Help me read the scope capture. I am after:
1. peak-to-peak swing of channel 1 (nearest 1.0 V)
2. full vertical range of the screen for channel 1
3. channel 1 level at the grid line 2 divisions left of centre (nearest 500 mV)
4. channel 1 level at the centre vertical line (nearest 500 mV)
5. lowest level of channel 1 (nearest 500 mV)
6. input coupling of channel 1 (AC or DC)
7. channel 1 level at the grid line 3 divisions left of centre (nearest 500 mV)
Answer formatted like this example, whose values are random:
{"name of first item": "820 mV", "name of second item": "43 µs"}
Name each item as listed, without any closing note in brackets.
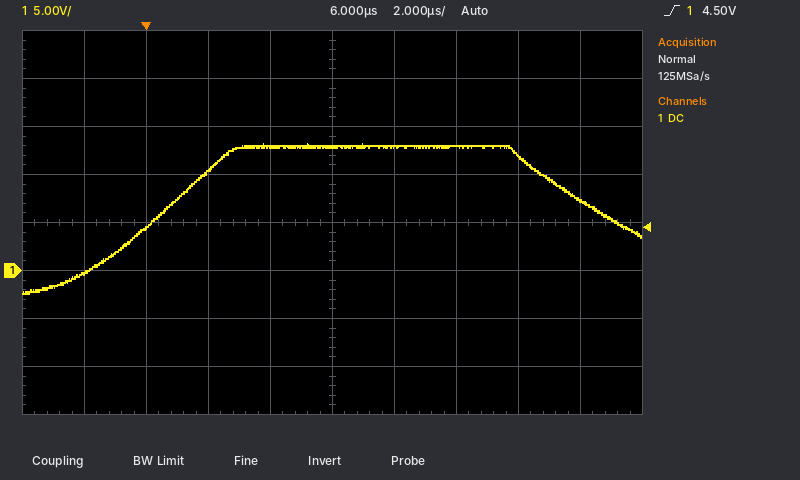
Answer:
{"peak-to-peak swing of channel 1": "16.0 V", "full vertical range of the screen for channel 1": "40 V", "channel 1 level at the grid line 2 divisions left of centre": "10.5 V", "channel 1 level at the centre vertical line": "13.0 V", "lowest level of channel 1": "-2.5 V", "input coupling of channel 1": "DC", "channel 1 level at the grid line 3 divisions left of centre": "4.5 V"}
